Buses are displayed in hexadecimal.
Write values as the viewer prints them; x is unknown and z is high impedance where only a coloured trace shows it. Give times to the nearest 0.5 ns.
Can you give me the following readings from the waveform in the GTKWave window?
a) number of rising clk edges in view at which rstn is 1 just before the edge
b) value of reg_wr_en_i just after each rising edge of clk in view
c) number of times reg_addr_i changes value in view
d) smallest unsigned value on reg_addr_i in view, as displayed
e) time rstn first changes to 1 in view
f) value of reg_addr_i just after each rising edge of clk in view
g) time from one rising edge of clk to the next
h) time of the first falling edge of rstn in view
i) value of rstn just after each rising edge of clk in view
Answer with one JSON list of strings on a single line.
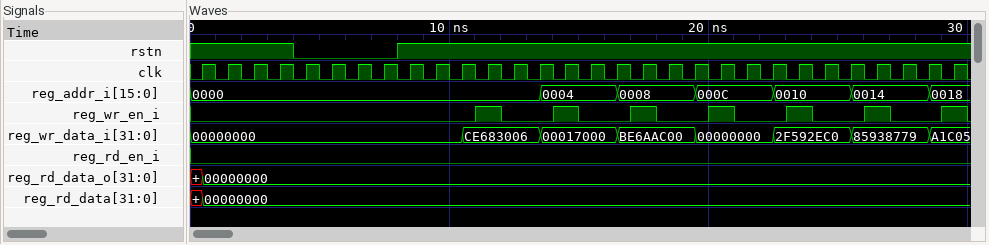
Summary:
["26", "0 0 0 0 0 0 0 0 0 0 0 1 0 0 1 0 0 1 0 0 1 0 0 1 0 0 1 0 0 1", "6", "0000", "8 ns", "0000, 0000, 0000, 0000, 0000, 0000, 0000, 0000, 0000, 0000, 0000, 0000, 0000, 0004, 0004, 0004, 0008, 0008, 0008, 000C, 000C, 000C, 0010, 0010, 0010, 0014, 0014, 0014, 0018, 0018", "1 ns", "4 ns", "1 1 1 1 0 0 0 0 1 1 1 1 1 1 1 1 1 1 1 1 1 1 1 1 1 1 1 1 1 1"]
